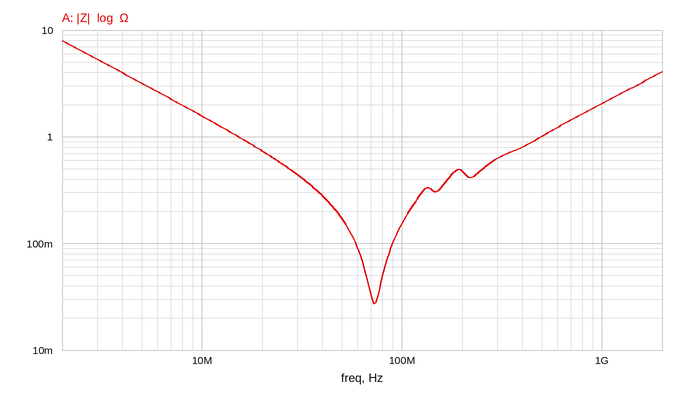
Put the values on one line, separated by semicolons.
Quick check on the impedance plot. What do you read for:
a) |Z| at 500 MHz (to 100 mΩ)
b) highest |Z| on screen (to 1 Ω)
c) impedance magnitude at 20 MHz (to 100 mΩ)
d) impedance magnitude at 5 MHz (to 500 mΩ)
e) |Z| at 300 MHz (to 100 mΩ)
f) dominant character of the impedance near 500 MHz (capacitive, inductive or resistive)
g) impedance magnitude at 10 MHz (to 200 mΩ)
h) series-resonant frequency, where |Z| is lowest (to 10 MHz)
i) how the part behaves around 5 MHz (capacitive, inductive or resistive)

1.0 Ω; 8 Ω; 700 mΩ; 3.0 Ω; 600 mΩ; inductive; 1.6 Ω; 70 MHz; capacitive
